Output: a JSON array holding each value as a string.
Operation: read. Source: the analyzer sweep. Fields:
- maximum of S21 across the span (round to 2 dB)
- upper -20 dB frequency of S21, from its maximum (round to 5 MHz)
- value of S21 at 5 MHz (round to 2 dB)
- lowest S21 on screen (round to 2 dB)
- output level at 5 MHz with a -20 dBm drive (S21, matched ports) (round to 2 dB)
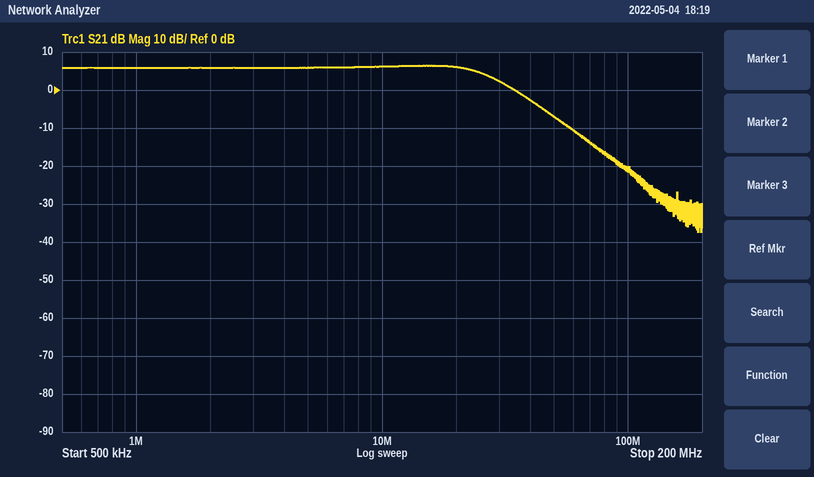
["6 dB", "70 MHz", "6 dB", "-38 dB", "-14 dBm"]
